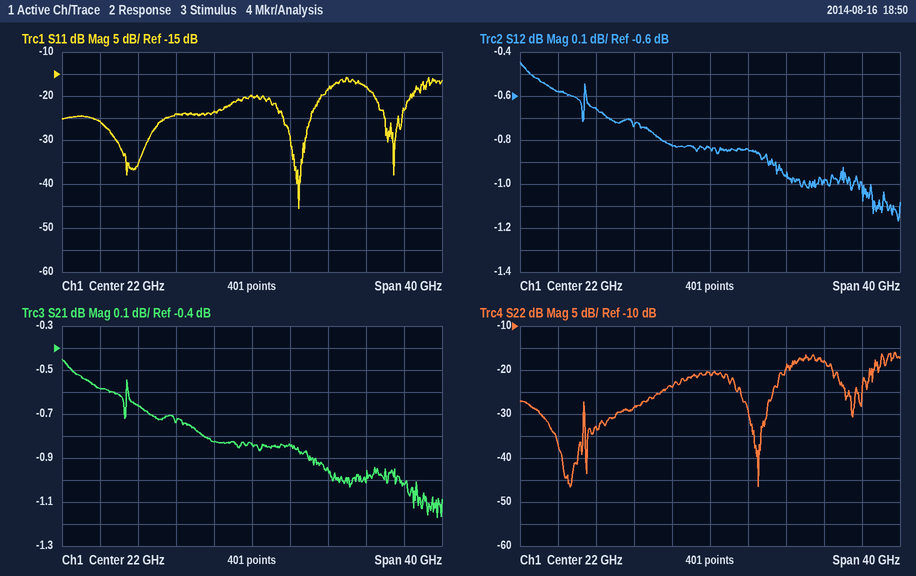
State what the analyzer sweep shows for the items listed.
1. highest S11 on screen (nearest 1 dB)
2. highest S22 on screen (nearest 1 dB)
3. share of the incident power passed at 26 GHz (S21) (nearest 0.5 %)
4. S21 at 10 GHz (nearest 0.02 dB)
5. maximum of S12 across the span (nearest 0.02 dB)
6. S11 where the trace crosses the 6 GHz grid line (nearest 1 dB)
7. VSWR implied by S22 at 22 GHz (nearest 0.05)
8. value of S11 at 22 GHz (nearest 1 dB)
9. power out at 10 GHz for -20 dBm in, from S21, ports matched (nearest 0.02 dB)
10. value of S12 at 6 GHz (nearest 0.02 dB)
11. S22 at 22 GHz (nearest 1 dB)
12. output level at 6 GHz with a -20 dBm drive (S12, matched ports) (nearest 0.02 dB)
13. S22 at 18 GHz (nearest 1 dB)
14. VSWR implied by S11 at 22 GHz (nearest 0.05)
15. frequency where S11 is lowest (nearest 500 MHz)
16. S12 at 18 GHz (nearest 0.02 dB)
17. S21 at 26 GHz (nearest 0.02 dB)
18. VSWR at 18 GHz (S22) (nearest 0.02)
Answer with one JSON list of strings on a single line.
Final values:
["-16 dB", "-16 dB", "82.5 %", "-0.66 dB", "-0.44 dB", "-26 dB", "1.20", "-20 dB", "-20.66 dBm", "-0.58 dB", "-21 dB", "-20.58 dBm", "-24 dB", "1.20", "27.0 GHz", "-0.82 dB", "-0.84 dB", "1.14"]
